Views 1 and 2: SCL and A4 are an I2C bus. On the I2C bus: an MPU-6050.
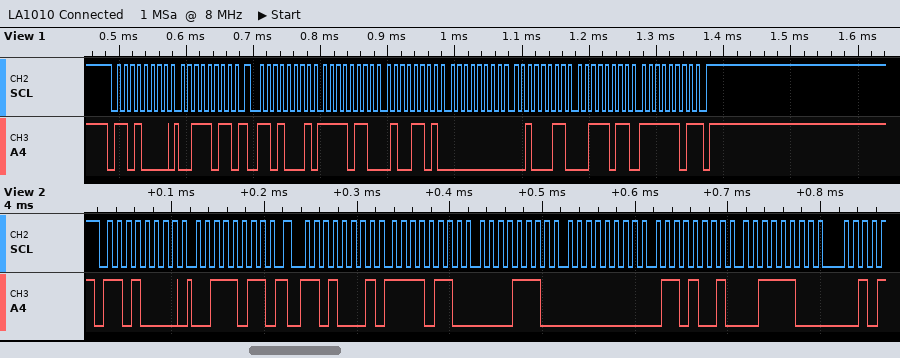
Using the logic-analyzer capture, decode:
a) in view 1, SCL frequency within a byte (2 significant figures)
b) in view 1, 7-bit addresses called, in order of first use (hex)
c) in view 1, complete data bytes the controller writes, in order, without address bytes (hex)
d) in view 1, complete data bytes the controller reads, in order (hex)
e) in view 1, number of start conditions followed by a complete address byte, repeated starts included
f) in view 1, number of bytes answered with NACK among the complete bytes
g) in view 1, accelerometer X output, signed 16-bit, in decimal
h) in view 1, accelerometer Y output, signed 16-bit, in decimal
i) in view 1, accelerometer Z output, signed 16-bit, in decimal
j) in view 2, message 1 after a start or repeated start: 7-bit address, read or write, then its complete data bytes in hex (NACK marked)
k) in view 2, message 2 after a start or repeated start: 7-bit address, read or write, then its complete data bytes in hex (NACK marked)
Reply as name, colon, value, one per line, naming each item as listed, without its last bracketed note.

in view 1, SCL frequency within a byte: 100 kHz
in view 1, 7-bit addresses called, in order of first use: 0x68
in view 1, complete data bytes the controller writes, in order, without address bytes: 3B
in view 1, complete data bytes the controller reads, in order: F6 4D 00 23 3B FD
in view 1, number of start conditions followed by a complete address byte, repeated starts included: 2
in view 1, number of bytes answered with NACK among the complete bytes: 1
in view 1, accelerometer X output, signed 16-bit, in decimal: -2483
in view 1, accelerometer Y output, signed 16-bit, in decimal: 35
in view 1, accelerometer Z output, signed 16-bit, in decimal: 15357
in view 2, message 1 after a start or repeated start: 7-bit address, read or write, then its complete data bytes in hex: 0x68 write: 3B
in view 2, message 2 after a start or repeated start: 7-bit address, read or write, then its complete data bytes in hex: 0x68 read: F6 0E 00 69 3C
